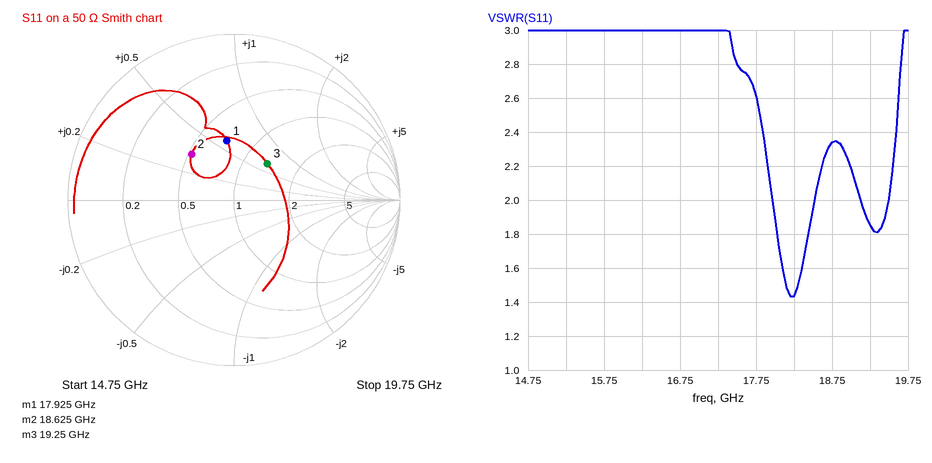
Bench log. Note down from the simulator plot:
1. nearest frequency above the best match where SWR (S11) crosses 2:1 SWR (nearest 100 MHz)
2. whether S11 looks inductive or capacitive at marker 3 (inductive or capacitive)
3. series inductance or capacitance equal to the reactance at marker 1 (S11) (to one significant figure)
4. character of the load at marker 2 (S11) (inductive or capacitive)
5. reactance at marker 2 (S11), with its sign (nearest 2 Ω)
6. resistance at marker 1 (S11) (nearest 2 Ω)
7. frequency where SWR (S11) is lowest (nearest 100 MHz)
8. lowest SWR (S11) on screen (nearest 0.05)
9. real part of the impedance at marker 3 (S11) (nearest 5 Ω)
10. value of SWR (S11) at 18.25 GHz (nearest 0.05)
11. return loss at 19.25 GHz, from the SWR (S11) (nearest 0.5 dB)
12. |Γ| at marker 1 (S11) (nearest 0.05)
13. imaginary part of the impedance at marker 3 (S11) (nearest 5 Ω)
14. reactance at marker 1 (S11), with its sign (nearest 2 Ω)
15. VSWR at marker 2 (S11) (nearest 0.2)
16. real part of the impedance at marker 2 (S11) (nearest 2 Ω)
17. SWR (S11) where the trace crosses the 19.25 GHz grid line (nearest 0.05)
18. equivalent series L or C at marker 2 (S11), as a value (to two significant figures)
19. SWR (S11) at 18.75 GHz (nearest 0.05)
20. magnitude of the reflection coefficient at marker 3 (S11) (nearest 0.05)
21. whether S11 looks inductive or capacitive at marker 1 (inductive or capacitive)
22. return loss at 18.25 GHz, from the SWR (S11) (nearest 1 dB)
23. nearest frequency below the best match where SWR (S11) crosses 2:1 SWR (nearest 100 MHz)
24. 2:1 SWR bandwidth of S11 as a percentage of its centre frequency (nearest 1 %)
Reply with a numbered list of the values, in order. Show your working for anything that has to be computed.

1. 18.5 GHz
2. inductive
3. L = 30 Ω/(2π × 17.925 GHz) ≈ 266 pH, so 300 pH to one significant figure
4. inductive
5. +16 Ω
6. 36 Ω
7. 18.2 GHz
8. 1.45
9. 65 Ω
10. 1.45
11. −20 log10((1.85 − 1)/(1.85 + 1)) ≈ 10.5 dB
12. 0.35
13. +30 Ω
14. +30 Ω
15. 2.2
16. 26 Ω
17. 1.85
18. L = 16 Ω/(2π × 18.625 GHz) ≈ 137 pH, so 140 pH to two significant figures
19. 2.35
20. 0.30
21. inductive
22. −20 log10((1.45 − 1)/(1.45 + 1)) ≈ 15 dB
23. 18.0 GHz
24. 500 MHz / 18.25 GHz ≈ 3 %
